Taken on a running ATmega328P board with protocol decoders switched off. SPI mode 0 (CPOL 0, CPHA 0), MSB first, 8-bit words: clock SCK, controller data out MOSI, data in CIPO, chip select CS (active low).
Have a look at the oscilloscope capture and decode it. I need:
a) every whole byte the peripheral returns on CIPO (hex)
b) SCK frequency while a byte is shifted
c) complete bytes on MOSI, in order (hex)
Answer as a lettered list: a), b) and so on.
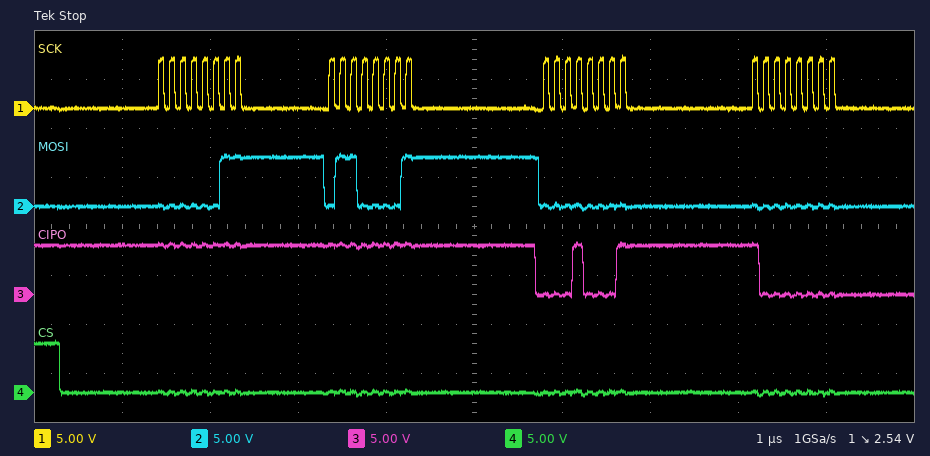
a) 0xFF 0xFF 0x11 0x80
b) 8 MHz
c) 0x03 0x61 0x00 0x00
